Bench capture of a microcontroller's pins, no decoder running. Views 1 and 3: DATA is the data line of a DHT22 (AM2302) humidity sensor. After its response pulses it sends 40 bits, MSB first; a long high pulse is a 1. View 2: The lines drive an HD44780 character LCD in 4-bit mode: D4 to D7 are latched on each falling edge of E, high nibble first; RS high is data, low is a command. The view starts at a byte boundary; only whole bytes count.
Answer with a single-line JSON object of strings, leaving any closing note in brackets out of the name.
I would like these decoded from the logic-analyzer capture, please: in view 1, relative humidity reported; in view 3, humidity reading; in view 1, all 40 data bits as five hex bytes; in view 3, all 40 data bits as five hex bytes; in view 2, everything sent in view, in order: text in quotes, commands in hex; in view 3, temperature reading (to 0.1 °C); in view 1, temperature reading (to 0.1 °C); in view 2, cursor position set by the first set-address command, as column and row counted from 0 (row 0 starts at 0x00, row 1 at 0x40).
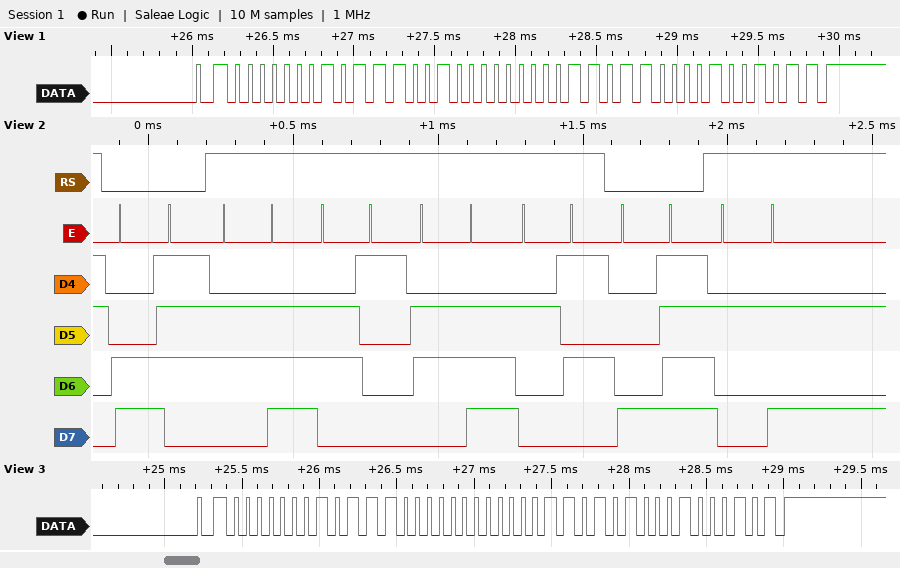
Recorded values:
{"in view 1, relative humidity reported": "37.0 %", "in view 3, humidity reading": "36.8 %", "in view 1, all 40 data bits as five hex bytes": "01 72 00 D8 4B", "in view 3, all 40 data bits as five hex bytes": "01 70 00 D4 45", "in view 2, everything sent in view, in order: text in quotes, commands in hex": "0xC7 \"nan%\" 0x8F \"*\"", "in view 3, temperature reading": "21.2 °C", "in view 1, temperature reading": "21.6 °C", "in view 2, cursor position set by the first set-address command, as column and row counted from 0": "column 7, row 1"}
